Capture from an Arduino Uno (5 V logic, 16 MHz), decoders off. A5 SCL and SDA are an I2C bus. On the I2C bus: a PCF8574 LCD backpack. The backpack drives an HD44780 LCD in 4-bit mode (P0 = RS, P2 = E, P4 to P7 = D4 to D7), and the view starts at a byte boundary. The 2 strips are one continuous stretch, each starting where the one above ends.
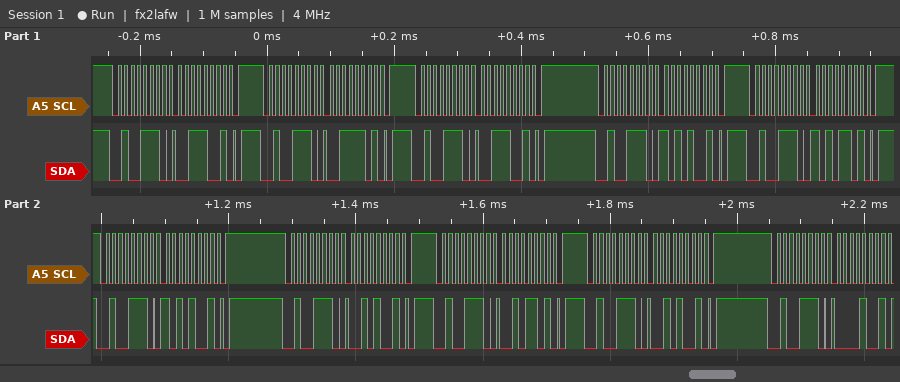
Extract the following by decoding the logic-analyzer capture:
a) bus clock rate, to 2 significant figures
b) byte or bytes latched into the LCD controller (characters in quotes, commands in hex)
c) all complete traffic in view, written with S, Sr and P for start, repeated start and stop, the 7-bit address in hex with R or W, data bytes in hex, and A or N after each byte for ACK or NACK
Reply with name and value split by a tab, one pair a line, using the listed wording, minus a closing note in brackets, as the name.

bus clock rate, to 2 significant figures	100 kHz
byte or bytes latched into the LCD controller	':'
all complete traffic in view, written with S, Sr and P for start, repeated start and stop, the 7-bit address in hex with R or W, data bytes in hex, and A or N after each byte for ACK or NACK	S 27W A 39 A P S 27W A 3D A P S 27W A 39 A P S 27W A A9 A P S 27W A AD A P S 27W A A9 A P S 27W A 29 A P S 27W A 2D A P S 27W A 29 A P S 27W A 09 A
